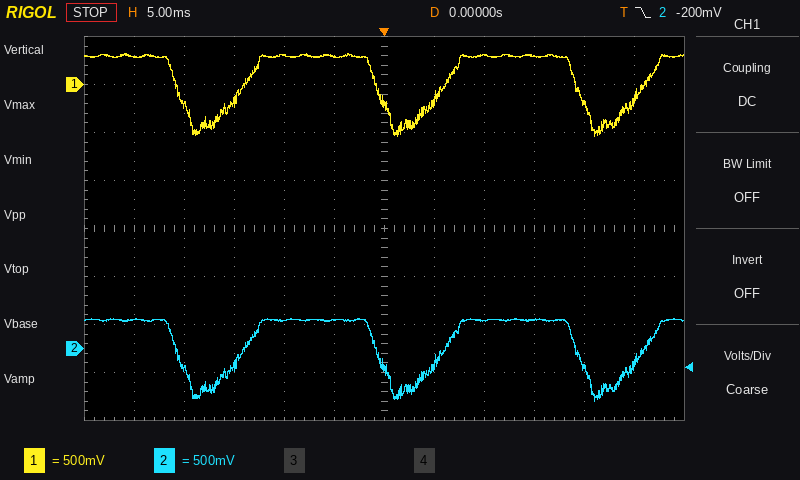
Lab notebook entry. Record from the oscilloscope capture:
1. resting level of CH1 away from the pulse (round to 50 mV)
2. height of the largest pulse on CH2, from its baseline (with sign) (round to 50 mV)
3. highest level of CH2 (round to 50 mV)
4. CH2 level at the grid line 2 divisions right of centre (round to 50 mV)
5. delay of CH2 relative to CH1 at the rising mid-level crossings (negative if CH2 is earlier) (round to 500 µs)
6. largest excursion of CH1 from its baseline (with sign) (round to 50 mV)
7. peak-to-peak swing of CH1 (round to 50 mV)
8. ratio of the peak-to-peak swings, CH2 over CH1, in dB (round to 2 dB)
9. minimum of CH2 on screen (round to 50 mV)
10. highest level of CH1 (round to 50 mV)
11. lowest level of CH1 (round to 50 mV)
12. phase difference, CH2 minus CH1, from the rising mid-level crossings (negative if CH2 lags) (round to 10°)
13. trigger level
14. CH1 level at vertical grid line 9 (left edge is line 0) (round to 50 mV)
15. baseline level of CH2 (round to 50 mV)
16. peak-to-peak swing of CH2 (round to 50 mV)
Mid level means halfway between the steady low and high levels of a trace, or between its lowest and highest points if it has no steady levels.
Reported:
300 mV
-850 mV
300 mV
300 mV
0.0 ms
-850 mV
850 mV
0 dB
-550 mV
300 mV
-550 mV
0°
-200 mV
300 mV
300 mV
850 mV
